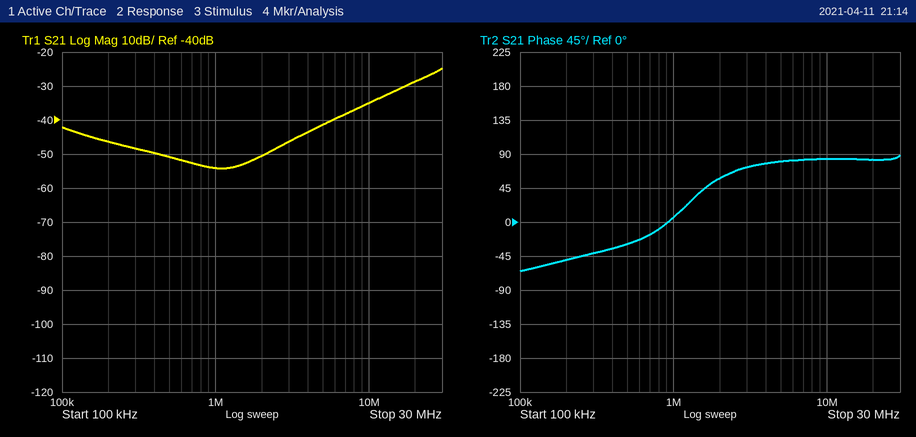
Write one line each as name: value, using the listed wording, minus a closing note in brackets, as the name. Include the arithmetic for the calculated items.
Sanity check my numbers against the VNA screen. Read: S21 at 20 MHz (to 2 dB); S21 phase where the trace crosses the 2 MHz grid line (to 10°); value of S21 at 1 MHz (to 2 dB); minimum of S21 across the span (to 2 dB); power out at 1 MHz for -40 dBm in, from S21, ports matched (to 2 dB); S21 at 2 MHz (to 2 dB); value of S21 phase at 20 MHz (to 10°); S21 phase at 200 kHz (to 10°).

S21 at 20 MHz: -28 dB
S21 phase where the trace crosses the 2 MHz grid line: 60°
value of S21 at 1 MHz: -54 dB
minimum of S21 across the span: -54 dB
power out at 1 MHz for -40 dBm in, from S21, ports matched: -40 dBm + (-54 dB) = -94 dBm
S21 at 2 MHz: -50 dB
value of S21 phase at 20 MHz: 80°
S21 phase at 200 kHz: -50°
